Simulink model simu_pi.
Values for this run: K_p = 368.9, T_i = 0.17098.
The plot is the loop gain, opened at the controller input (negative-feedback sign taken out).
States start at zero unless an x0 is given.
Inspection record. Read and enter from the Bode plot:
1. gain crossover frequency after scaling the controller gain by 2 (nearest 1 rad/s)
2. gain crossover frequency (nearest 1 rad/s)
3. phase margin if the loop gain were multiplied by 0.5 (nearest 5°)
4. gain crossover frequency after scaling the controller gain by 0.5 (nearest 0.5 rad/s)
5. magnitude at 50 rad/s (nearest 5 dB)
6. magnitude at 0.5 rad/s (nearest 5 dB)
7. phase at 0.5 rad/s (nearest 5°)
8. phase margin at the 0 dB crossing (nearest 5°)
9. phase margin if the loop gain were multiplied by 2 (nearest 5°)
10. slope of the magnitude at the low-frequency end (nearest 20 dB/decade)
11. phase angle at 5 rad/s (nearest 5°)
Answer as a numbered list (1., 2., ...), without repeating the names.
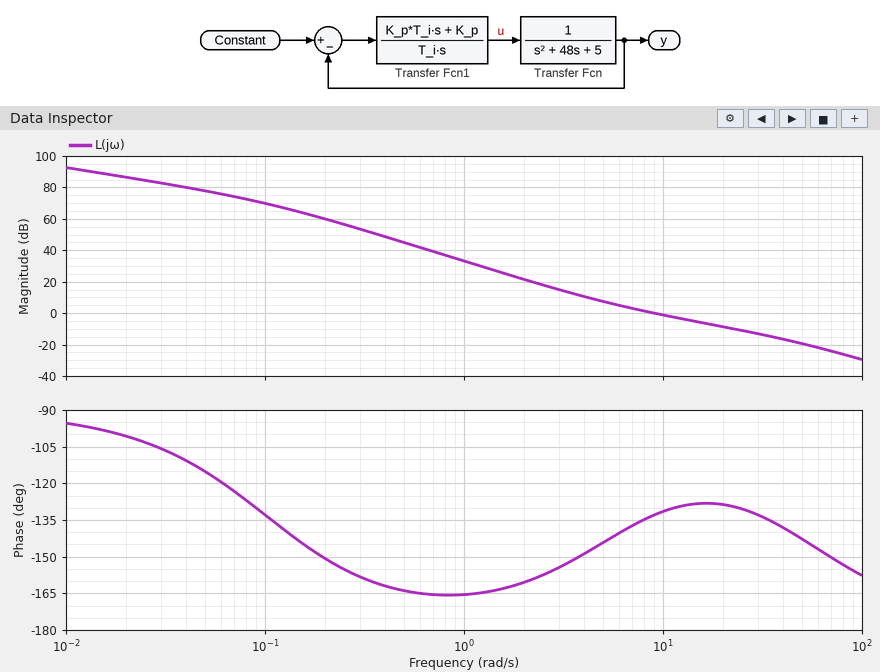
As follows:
1. 16 rad/s
2. 9 rad/s
3. 40°
4. 5.5 rad/s
5. -20 dB
6. 45 dB
7. -165°
8. 45°
9. 50°
10. -20 dB/decade
11. -145°
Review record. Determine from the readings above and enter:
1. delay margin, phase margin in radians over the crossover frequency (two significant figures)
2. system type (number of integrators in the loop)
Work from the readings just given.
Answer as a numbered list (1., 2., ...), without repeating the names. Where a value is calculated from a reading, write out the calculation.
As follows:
1. 45 × π / 180 / 9 = 0.087 s
2. 1
